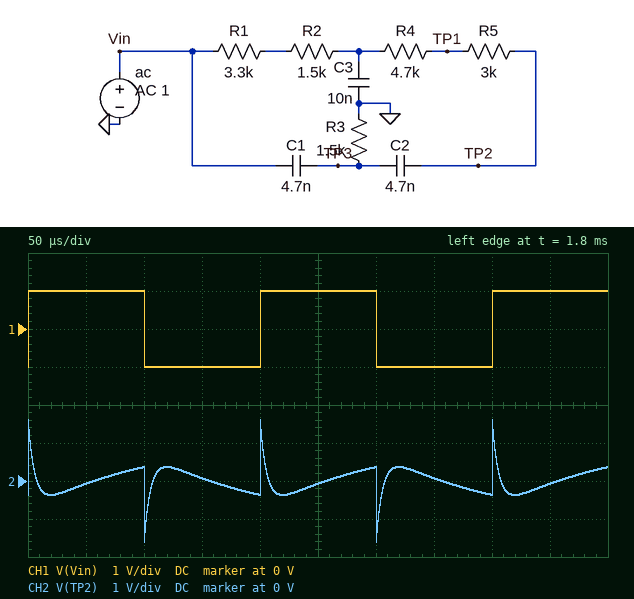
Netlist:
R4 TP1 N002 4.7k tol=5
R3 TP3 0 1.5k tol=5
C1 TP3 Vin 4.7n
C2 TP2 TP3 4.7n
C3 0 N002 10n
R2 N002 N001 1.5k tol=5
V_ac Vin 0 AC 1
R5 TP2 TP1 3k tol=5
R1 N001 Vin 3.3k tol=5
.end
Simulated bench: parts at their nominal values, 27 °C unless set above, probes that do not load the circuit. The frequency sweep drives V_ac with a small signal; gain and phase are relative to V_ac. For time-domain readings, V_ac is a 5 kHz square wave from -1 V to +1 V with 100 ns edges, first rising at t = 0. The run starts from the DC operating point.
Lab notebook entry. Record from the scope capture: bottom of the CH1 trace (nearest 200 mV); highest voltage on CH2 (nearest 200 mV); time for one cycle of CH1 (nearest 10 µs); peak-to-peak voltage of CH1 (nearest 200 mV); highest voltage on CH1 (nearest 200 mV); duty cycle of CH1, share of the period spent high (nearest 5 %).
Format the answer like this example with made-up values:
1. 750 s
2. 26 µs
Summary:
1. -1.0 V
2. 1.6 V
3. 200 µs
4. 2.0 V
5. 1.0 V
6. 50 %
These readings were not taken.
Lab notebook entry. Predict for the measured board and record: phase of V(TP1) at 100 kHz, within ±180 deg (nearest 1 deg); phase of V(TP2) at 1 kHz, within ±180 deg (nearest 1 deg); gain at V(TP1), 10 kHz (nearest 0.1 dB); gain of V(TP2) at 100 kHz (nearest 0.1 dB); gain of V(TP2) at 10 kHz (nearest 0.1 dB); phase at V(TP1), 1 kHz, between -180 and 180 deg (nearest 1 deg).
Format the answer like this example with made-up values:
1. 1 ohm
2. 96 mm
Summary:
1. 16 deg
2. -35 deg
3. -24.8 dB
4. -0.4 dB
5. -13.9 dB
6. -30 deg
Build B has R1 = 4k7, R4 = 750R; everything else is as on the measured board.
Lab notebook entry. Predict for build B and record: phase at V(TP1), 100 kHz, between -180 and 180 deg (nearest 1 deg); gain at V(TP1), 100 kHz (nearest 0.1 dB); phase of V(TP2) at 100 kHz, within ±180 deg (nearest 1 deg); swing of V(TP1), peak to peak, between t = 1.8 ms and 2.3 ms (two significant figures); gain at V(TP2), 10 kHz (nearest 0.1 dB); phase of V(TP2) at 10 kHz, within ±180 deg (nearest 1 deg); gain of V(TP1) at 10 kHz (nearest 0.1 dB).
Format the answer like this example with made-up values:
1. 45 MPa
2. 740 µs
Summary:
1. 7 deg
2. -14.5 dB
3. 22 deg
4. 970 mV
5. -19.4 dB
6. 109 deg
7. -16.9 dB
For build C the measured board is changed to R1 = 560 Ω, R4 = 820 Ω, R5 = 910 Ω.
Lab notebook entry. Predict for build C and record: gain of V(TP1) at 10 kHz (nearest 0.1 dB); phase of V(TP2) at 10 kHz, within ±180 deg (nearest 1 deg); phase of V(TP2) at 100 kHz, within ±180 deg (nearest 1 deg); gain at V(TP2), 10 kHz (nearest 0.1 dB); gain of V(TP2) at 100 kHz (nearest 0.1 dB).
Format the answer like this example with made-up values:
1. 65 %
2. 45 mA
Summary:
1. -9.2 dB
2. -64 deg
3. 32 deg
4. -12.5 dB
5. -1.6 dB
